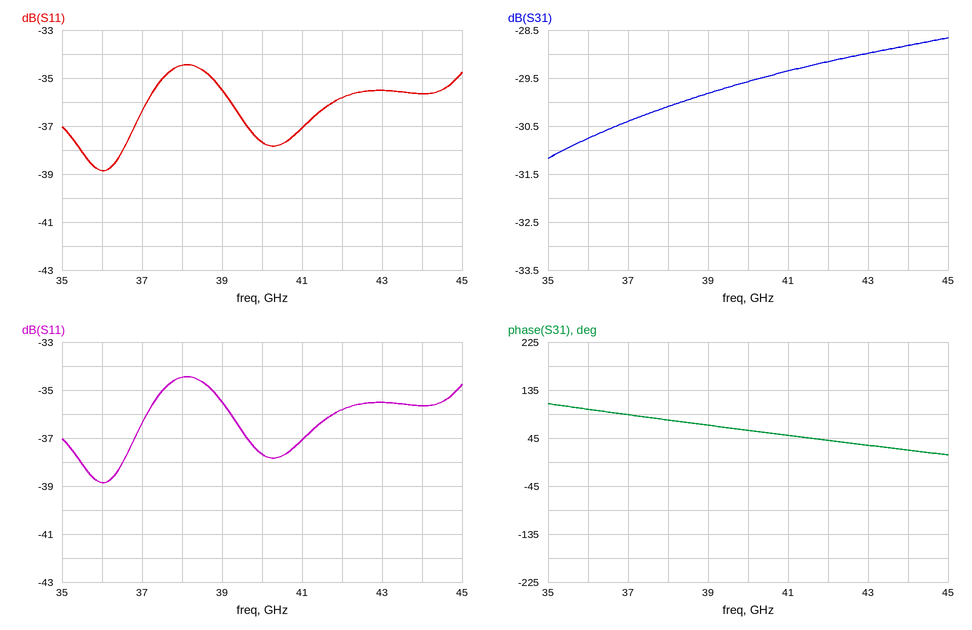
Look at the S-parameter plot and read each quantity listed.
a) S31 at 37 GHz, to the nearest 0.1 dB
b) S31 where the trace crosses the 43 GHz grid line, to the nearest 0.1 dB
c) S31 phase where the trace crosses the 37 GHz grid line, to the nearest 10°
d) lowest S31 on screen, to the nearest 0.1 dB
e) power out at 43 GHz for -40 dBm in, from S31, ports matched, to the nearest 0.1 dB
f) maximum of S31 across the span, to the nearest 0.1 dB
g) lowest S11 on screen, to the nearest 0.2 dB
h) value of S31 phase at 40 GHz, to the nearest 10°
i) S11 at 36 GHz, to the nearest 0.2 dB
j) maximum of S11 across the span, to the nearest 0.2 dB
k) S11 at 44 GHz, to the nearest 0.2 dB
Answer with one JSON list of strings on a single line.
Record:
["-30.4 dB", "-29.0 dB", "90°", "-31.2 dB", "-69.0 dBm", "-28.7 dB", "-38.8 dB", "60°", "-38.8 dB", "-34.4 dB", "-35.6 dB"]
